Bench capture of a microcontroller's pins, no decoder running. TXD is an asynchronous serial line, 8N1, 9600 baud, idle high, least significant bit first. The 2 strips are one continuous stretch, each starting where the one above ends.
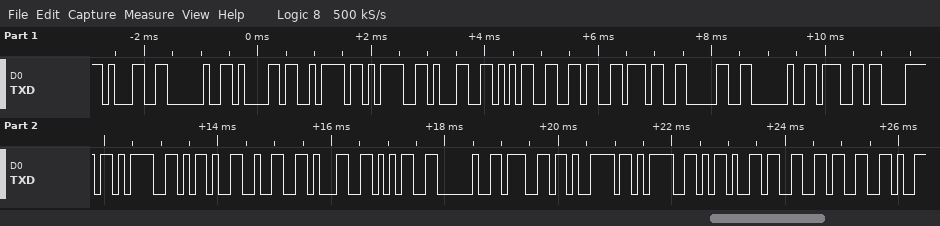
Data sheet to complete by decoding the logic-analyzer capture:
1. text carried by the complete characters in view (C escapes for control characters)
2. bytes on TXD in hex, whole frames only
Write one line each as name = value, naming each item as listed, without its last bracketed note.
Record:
text carried by the complete characters in view = "1 az=15670 gx=-215 gy=-33"
bytes on TXD in hex, whole frames only = 31 20 61 7A 3D 31 35 36 37 30 20 67 78 3D 2D 32 31 35 20 67 79 3D 2D 33 33
